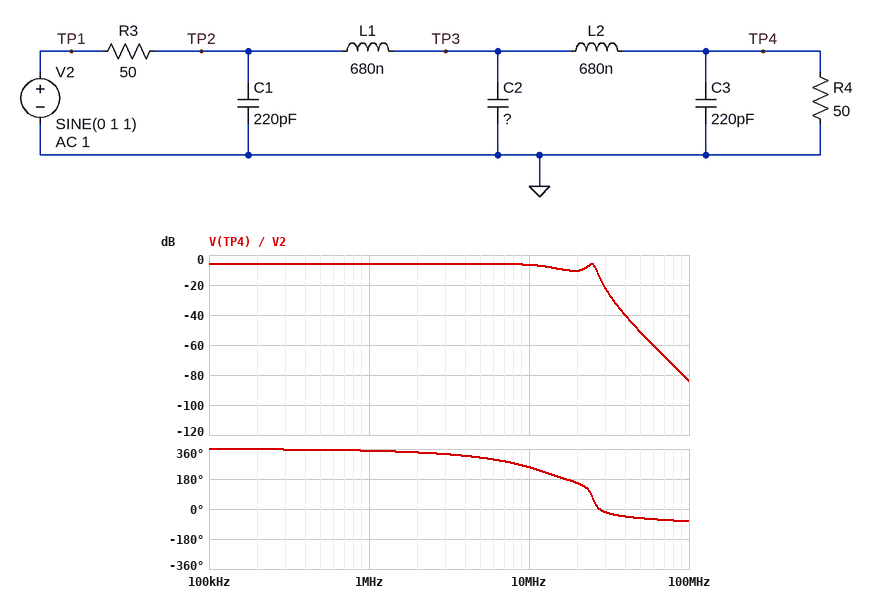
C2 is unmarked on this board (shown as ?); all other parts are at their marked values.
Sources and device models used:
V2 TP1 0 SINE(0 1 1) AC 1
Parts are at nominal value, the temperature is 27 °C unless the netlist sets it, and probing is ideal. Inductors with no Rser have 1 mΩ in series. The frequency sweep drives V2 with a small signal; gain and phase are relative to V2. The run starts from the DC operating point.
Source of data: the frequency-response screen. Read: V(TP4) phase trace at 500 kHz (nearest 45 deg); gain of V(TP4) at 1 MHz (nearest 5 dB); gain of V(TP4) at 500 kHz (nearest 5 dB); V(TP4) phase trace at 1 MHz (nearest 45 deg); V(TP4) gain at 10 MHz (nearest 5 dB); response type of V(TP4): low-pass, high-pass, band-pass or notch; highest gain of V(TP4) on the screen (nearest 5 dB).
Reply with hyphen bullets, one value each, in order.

- 360 deg
- -5 dB
- -5 dB
- 360 deg
- -5 dB
- low-pass
- -5 dB
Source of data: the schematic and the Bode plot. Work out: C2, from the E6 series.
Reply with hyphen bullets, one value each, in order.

- 150 pF
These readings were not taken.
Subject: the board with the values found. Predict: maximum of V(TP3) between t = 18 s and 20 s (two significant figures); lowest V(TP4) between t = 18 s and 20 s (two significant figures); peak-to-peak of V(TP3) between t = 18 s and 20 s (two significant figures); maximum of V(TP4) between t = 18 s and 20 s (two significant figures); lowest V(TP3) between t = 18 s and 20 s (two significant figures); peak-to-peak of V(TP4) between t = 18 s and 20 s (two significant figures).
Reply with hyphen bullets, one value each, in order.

- 500 mV
- -500 mV
- 1.0 V
- 500 mV
- -500 mV
- 1.0 V
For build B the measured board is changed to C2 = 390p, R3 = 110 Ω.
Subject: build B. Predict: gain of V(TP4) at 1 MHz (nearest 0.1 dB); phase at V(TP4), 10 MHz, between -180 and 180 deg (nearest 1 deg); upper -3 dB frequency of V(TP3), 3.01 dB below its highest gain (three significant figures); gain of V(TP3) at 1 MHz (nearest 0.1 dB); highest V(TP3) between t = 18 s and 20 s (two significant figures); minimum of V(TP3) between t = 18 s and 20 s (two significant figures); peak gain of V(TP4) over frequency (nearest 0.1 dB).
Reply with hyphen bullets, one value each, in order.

- -10.1 dB
- -128 deg
- 19.4 MHz
- -10.2 dB
- 310 mV
- -310 mV
- -9.5 dB
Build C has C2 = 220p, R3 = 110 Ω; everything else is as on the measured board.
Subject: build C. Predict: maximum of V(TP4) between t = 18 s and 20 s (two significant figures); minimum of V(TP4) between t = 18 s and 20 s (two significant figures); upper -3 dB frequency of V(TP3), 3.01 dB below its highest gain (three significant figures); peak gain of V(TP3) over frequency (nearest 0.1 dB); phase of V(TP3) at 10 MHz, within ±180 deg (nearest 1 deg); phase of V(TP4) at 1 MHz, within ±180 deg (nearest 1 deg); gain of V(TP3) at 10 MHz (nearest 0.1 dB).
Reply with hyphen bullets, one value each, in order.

- 310 mV
- -310 mV
- 23.1 MHz
- -1.4 dB
- -52 deg
- -11 deg
- -10.1 dB
